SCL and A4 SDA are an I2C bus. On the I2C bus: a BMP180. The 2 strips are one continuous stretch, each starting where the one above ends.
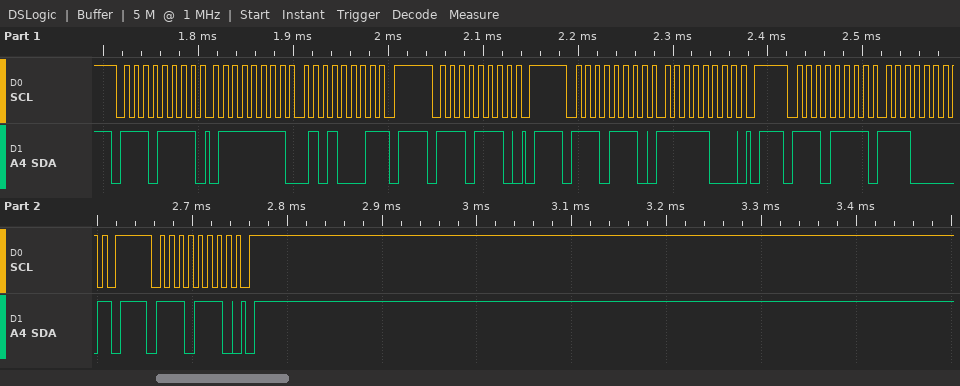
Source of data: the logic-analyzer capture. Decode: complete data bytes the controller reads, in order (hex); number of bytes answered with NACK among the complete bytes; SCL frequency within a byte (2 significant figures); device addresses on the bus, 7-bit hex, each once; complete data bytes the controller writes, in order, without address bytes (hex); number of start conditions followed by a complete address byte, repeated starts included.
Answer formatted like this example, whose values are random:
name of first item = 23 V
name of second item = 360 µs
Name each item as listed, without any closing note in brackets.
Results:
complete data bytes the controller reads, in order = 7F 51 E0
number of bytes answered with NACK among the complete bytes = 2
SCL frequency within a byte = 100 kHz
device addresses on the bus, 7-bit hex, each once = 0x77
complete data bytes the controller writes, in order, without address bytes = F8
number of start conditions followed by a complete address byte, repeated starts included = 5
